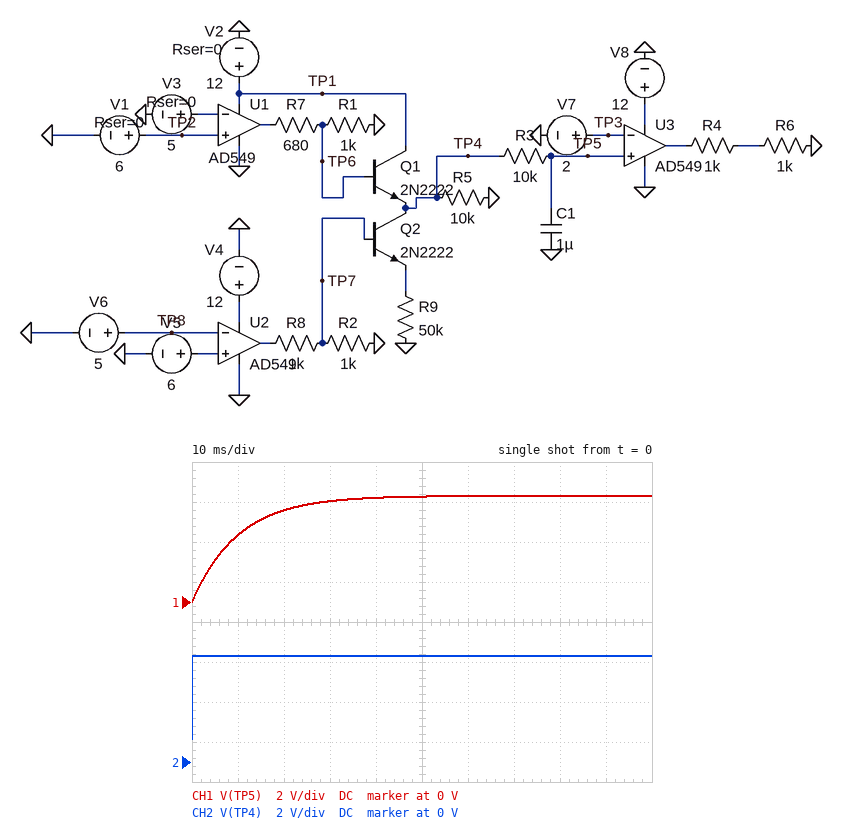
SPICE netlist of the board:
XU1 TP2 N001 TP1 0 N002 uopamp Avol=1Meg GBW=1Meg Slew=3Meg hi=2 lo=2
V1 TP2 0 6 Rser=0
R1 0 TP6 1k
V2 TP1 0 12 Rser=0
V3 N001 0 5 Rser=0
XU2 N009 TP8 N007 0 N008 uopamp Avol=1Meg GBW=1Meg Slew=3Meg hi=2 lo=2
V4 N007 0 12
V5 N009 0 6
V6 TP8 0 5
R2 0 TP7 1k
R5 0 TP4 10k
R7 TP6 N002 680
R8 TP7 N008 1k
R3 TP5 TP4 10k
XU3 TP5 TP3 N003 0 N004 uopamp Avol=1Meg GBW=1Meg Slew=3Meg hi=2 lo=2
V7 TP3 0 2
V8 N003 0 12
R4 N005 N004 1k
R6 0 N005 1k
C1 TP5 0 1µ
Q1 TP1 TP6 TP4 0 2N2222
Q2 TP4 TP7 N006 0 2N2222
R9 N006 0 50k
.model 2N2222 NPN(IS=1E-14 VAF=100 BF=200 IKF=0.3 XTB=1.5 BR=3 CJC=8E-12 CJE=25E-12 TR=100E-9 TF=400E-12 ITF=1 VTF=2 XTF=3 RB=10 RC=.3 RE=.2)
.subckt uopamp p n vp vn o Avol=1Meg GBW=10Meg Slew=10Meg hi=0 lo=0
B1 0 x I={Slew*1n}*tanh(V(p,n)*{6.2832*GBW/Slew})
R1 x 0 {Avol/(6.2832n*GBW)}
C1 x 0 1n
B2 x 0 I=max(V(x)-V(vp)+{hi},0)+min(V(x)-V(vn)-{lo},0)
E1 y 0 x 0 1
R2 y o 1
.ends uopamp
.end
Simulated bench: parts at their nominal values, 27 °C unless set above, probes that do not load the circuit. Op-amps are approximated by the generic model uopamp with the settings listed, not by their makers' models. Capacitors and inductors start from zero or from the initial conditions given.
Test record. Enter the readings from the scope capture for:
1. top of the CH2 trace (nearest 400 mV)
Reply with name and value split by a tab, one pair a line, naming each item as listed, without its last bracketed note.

top of the CH2 trace	5.2 V
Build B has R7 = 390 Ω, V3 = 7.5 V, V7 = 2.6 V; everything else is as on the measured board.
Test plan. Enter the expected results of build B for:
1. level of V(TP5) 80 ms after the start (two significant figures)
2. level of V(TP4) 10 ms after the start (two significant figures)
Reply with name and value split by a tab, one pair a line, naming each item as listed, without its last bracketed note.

level of V(TP5) 80 ms after the start	4.1 V
level of V(TP4) 10 ms after the start	4.0 V
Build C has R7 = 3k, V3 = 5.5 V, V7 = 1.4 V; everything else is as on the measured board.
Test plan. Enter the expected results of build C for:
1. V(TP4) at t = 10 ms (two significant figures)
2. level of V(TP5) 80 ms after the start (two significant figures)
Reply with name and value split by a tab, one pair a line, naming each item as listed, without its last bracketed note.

V(TP4) at t = 10 ms	4.0 V
level of V(TP5) 80 ms after the start	4.1 V
